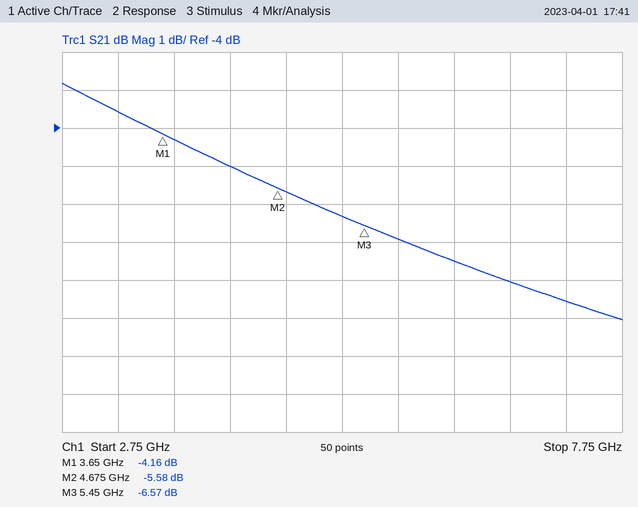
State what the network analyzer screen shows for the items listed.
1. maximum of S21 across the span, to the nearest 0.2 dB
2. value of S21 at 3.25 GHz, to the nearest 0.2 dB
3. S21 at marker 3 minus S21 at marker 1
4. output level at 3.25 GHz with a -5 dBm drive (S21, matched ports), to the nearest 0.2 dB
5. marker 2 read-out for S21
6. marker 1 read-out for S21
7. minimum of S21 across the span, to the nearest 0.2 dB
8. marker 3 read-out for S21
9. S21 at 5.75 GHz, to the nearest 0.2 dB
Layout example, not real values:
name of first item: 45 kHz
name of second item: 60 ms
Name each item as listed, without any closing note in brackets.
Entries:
maximum of S21 across the span, to the nearest 0.2 dB: -2.8 dB
value of S21 at 3.25 GHz, to the nearest 0.2 dB: -3.6 dB
S21 at marker 3 minus S21 at marker 1: -2.41 dB
output level at 3.25 GHz with a -5 dBm drive (S21, matched ports), to the nearest 0.2 dB: -8.6 dBm
marker 2 read-out for S21: -5.58 dB
marker 1 read-out for S21: -4.16 dB
minimum of S21 across the span, to the nearest 0.2 dB: -9.0 dB
marker 3 read-out for S21: -6.57 dB
S21 at 5.75 GHz, to the nearest 0.2 dB: -7.0 dB
